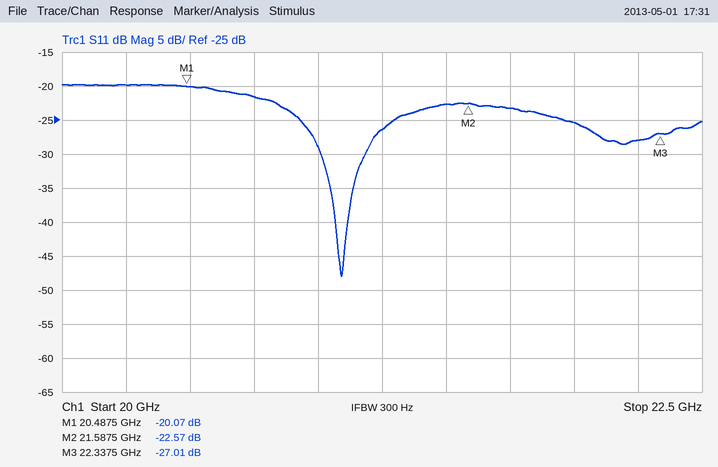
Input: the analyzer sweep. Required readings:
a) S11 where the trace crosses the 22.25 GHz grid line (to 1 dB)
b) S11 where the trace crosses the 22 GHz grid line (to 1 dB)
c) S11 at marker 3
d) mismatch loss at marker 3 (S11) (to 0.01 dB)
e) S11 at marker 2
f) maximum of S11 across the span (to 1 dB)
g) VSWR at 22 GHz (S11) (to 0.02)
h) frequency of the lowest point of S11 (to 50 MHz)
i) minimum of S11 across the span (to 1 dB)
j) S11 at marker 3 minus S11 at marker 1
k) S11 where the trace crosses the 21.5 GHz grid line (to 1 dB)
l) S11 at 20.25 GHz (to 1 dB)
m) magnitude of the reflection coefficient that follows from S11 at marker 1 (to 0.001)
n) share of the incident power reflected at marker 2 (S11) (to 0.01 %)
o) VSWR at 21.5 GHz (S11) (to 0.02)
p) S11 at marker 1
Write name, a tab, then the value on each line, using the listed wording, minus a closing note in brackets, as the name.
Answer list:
S11 where the trace crosses the 22.25 GHz grid line	-28 dB
S11 where the trace crosses the 22 GHz grid line	-25 dB
S11 at marker 3	-27.01 dB
mismatch loss at marker 3 (S11)	0.01 dB
S11 at marker 2	-22.57 dB
maximum of S11 across the span	-20 dB
VSWR at 22 GHz (S11)	1.12
frequency of the lowest point of S11	21.10 GHz
minimum of S11 across the span	-48 dB
S11 at marker 3 minus S11 at marker 1	-6.94 dB
S11 where the trace crosses the 21.5 GHz grid line	-23 dB
S11 at 20.25 GHz	-20 dB
magnitude of the reflection coefficient that follows from S11 at marker 1	0.099
share of the incident power reflected at marker 2 (S11)	0.55 %
VSWR at 21.5 GHz (S11)	1.16
S11 at marker 1	-20.07 dB
